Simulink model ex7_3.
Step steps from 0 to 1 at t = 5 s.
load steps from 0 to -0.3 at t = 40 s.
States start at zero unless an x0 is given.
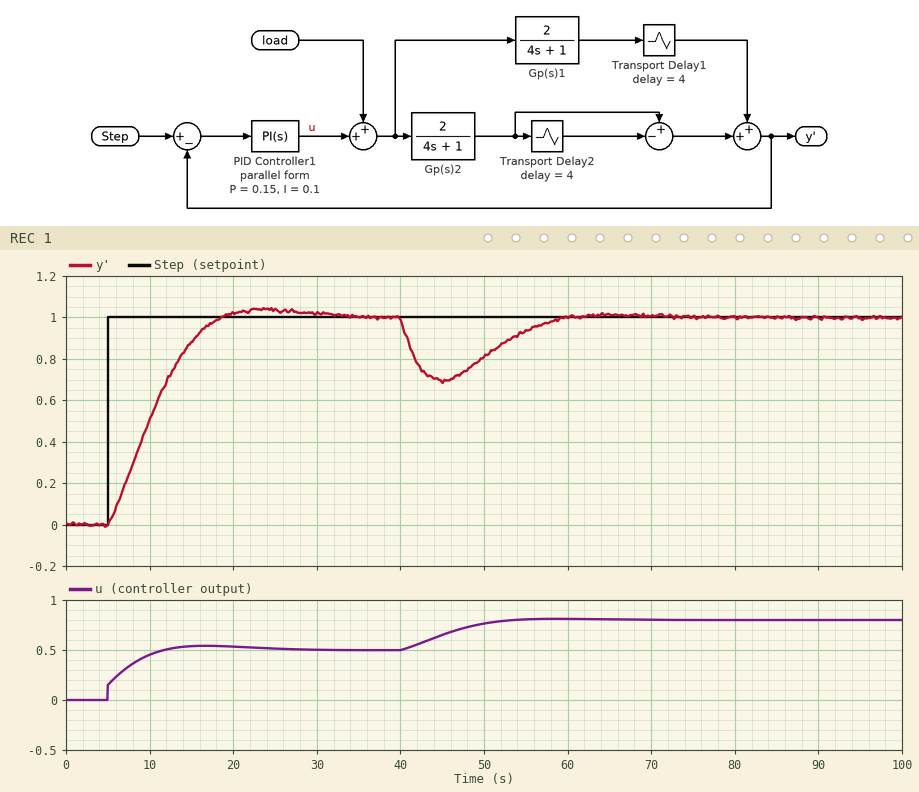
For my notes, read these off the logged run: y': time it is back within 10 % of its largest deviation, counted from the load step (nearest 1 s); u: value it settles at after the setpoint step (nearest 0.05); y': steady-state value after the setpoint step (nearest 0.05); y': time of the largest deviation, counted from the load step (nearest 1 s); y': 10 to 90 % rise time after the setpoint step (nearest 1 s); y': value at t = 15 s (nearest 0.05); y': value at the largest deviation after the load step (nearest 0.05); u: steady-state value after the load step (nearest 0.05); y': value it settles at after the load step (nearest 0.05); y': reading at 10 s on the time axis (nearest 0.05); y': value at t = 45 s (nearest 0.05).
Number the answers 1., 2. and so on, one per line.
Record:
1. 17 s
2. 0.50
3. 1.00
4. 5 s
5. 9 s
6. 0.90
7. 0.70
8. 0.80
9. 1.00
10. 0.50
11. 0.70
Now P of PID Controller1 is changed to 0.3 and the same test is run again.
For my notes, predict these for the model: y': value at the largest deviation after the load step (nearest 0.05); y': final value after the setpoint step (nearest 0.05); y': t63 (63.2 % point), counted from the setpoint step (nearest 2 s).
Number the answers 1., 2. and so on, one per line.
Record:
1. 0.75
2. 1.00
3. 6 s
